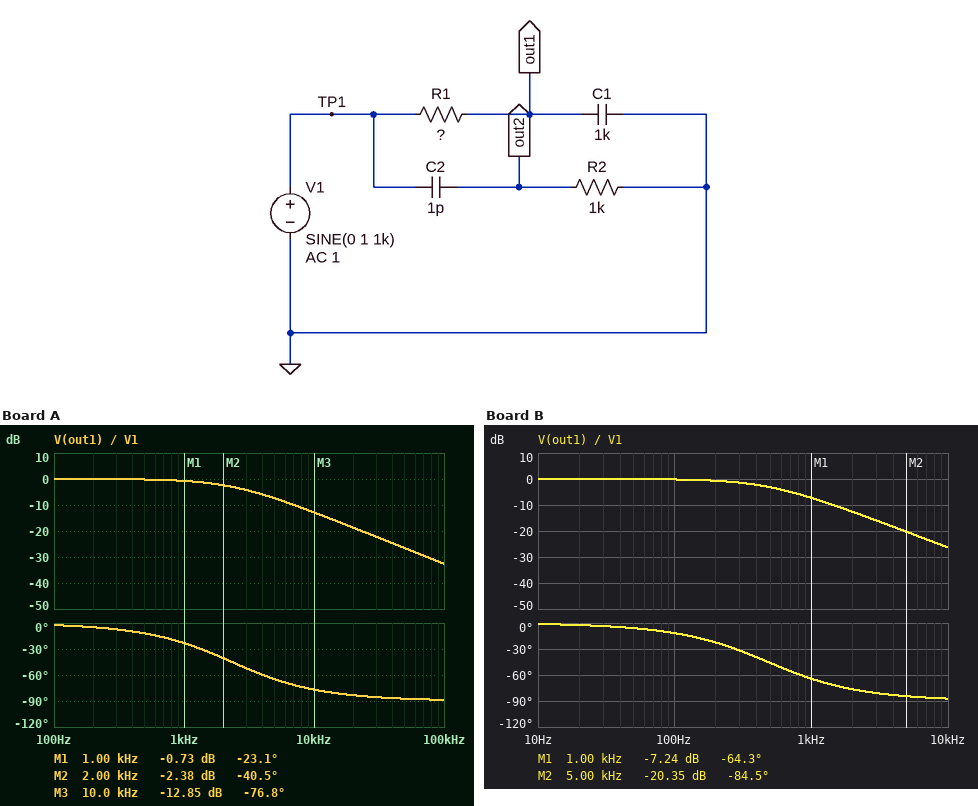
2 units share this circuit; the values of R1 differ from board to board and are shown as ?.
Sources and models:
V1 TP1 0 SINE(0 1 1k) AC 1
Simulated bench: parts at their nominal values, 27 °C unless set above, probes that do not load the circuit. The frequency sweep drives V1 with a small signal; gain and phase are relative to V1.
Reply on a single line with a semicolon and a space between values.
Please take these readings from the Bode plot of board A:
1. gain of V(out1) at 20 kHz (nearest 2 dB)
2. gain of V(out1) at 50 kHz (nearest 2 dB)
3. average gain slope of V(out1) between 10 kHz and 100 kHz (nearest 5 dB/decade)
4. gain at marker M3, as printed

-18 dB; -26 dB; -20 dB/decade; -12.85 dB
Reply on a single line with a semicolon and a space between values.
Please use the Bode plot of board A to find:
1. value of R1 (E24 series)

68 nΩ
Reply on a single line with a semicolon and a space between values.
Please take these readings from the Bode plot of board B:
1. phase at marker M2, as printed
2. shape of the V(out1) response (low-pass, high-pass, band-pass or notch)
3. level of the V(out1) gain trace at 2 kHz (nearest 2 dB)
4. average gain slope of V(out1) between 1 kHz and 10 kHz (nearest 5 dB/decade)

-84.5 deg; low-pass; -12 dB; -20 dB/decade
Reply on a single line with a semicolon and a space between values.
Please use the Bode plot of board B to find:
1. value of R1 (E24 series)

330 nΩ
